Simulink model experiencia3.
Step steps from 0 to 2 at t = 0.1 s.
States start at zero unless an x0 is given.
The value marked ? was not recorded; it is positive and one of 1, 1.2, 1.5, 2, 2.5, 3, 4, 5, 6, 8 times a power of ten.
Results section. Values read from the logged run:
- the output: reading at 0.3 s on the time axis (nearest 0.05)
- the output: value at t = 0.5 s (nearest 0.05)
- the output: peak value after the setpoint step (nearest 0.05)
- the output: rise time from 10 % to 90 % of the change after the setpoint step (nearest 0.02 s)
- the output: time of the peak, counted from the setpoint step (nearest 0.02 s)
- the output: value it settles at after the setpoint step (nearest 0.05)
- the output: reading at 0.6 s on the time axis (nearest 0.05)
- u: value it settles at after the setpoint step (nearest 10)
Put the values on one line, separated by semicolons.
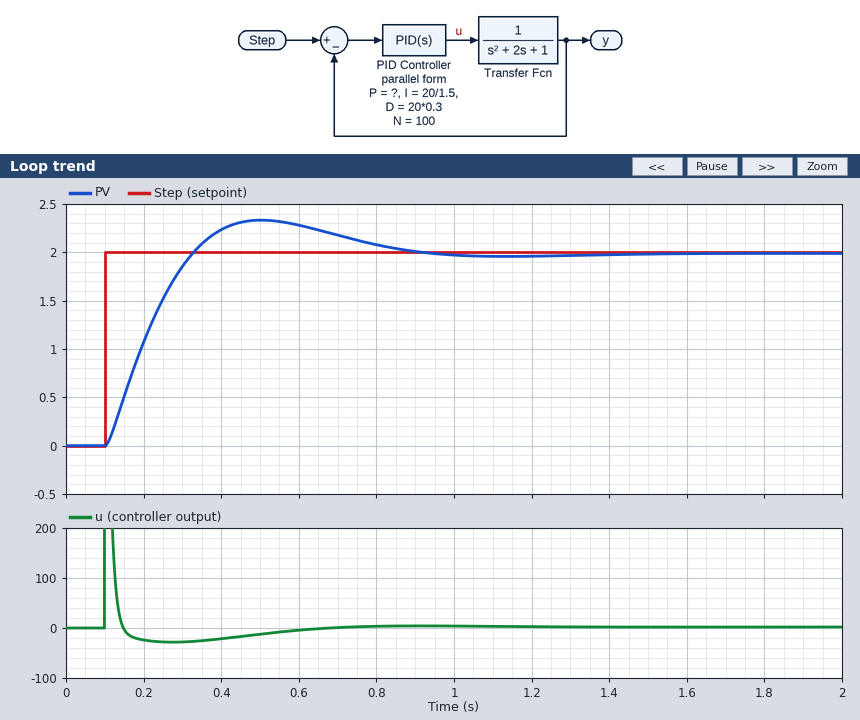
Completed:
1.85; 2.35; 2.35; 0.16 s; 0.40 s; 2.00; 2.30; 0
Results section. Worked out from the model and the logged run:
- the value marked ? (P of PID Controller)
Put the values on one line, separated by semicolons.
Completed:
40
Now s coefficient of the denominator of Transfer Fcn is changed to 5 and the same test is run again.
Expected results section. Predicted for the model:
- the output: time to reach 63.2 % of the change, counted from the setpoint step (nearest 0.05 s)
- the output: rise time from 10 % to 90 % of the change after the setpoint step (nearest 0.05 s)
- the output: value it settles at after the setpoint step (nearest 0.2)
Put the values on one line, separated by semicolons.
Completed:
0.15 s; 0.25 s; 2.0
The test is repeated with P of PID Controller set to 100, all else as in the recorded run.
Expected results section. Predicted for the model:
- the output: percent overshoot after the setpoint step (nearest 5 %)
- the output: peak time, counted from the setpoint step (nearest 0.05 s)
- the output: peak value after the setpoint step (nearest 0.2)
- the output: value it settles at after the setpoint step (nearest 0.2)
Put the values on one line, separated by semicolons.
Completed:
35 %; 0.25 s; 2.6; 2.0
